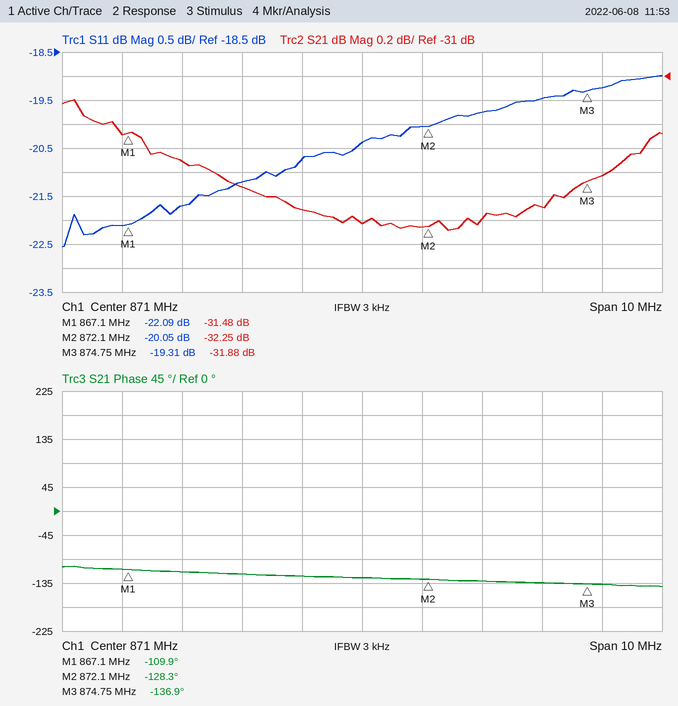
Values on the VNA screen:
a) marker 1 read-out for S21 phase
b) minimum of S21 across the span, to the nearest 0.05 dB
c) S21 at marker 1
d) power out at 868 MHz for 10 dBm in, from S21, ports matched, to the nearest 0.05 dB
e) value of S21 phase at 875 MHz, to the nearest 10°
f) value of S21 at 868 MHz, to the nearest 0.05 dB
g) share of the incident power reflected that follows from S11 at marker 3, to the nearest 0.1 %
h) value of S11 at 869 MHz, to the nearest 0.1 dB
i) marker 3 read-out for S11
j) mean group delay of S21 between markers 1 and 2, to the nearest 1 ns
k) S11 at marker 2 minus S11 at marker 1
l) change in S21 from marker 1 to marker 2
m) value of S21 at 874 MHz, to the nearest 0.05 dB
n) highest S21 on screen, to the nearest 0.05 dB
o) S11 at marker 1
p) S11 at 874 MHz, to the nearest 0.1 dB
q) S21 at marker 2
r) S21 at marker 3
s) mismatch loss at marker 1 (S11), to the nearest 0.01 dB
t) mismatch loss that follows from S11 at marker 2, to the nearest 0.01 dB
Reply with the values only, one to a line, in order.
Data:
-109.9°
-32.30 dB
-31.48 dB
-21.70 dBm
-140°
-31.70 dB
1.2 %
-21.2 dB
-19.31 dB
10 ns
2.04 dB
-0.77 dB
-32.10 dB
-31.20 dB
-22.09 dB
-19.5 dB
-32.25 dB
-31.88 dB
0.03 dB
0.04 dB
